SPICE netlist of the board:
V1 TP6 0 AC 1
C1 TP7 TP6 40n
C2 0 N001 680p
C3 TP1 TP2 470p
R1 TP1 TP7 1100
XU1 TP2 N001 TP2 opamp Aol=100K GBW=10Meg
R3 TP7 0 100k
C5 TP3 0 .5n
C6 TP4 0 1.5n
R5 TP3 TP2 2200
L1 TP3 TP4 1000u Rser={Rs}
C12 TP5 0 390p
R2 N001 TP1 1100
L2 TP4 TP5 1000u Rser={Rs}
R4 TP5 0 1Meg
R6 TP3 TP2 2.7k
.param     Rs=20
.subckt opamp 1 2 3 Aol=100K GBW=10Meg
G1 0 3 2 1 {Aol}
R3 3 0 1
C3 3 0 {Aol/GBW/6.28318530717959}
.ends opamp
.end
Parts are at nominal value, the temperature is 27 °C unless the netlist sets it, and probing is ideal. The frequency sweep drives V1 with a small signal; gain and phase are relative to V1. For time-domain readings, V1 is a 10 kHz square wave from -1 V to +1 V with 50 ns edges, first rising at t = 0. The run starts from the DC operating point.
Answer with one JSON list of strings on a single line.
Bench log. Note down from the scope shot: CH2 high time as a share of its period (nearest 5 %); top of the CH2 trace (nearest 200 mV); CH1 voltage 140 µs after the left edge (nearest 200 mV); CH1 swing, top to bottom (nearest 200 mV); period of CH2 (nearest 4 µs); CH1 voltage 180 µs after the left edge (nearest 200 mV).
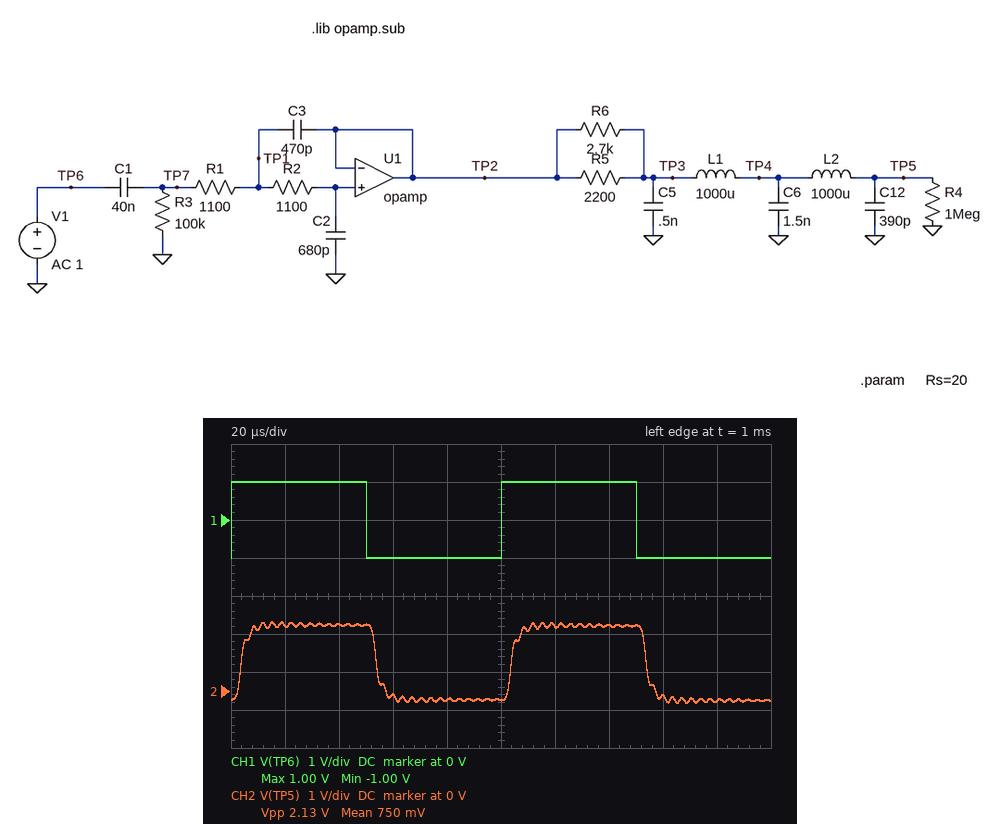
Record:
["50 %", "1.8 V", "1.0 V", "2.0 V", "100 µs", "-1.0 V"]
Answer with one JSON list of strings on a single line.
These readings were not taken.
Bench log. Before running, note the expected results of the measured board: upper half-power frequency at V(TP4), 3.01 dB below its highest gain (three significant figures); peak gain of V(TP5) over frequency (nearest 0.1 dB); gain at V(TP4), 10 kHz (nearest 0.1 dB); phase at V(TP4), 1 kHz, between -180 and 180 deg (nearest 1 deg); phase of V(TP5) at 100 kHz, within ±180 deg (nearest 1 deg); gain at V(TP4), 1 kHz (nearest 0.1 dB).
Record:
["60.8 kHz", "2.2 dB", "-0.3 dB", "1 deg", "-131 deg", "-0.2 dB"]
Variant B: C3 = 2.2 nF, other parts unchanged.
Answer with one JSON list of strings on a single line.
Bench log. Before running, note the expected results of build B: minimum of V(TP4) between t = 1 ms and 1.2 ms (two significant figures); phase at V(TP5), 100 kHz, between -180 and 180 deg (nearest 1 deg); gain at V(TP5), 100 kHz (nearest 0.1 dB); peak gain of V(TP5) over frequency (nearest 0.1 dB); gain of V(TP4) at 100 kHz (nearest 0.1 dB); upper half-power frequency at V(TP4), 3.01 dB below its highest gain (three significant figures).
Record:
["-260 mV", "-157 deg", "-2.8 dB", "-0.2 dB", "-4.3 dB", "86.4 kHz"]
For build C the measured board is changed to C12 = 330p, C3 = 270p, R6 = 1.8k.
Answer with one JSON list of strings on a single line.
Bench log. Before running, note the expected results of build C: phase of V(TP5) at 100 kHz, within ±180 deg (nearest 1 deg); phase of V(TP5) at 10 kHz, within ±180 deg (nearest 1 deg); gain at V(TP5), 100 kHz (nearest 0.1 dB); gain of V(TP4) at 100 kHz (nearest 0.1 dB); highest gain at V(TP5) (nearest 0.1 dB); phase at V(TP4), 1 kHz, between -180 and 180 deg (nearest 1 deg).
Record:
["-125 deg", "-14 deg", "-3.5 dB", "-4.7 dB", "4.4 dB", "1 deg"]
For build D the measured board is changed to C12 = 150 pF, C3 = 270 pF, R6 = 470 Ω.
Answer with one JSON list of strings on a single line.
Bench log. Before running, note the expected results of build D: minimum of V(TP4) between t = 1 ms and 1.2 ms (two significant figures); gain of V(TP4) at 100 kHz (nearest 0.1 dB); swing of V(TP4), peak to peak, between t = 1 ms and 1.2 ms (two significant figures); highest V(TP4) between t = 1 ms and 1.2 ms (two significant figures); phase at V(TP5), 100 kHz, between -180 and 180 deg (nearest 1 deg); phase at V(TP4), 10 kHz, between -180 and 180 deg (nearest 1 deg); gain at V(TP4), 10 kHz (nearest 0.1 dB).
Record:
["-720 mV", "2.3 dB", "2.9 V", "2.2 V", "-100 deg", "-8 deg", "-0.1 dB"]
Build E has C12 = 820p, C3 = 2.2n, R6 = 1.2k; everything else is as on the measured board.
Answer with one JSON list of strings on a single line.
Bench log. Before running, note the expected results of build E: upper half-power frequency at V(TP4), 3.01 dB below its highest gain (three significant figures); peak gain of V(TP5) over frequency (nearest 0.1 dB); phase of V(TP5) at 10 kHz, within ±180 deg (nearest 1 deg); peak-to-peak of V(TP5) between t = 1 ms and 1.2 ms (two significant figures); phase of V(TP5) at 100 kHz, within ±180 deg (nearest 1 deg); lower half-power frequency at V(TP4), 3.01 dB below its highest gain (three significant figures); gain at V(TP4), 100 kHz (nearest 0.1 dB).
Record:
["102 kHz", "1.3 dB", "-13 deg", "2.7 V", "-168 deg", "41.0 Hz", "-2.7 dB"]
